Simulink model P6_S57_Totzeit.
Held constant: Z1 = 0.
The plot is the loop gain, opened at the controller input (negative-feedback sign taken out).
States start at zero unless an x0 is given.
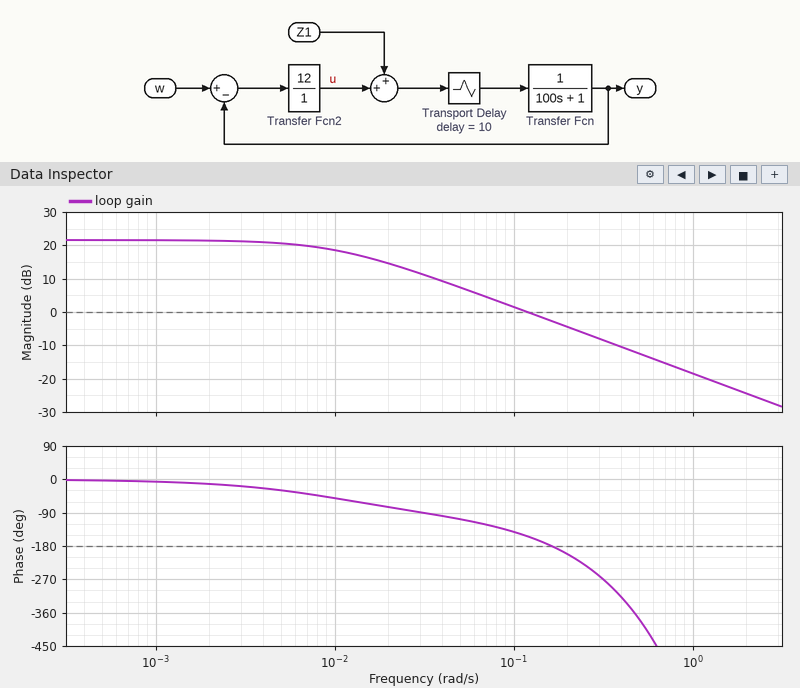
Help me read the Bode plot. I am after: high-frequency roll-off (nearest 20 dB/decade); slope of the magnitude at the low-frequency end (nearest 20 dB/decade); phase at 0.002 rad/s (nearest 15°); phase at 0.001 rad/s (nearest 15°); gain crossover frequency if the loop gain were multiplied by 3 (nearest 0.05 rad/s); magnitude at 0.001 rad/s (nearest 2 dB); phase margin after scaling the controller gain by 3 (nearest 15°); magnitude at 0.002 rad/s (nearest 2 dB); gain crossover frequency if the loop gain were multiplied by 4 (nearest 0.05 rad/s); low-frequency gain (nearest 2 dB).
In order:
-20 dB/decade
0 dB/decade
-15°
0°
0.35 rad/s
22 dB
-120°
22 dB
0.50 rad/s
22 dB
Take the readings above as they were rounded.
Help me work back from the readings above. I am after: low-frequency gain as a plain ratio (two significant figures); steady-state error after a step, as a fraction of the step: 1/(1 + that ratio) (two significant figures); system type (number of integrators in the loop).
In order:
13
0.071
0
